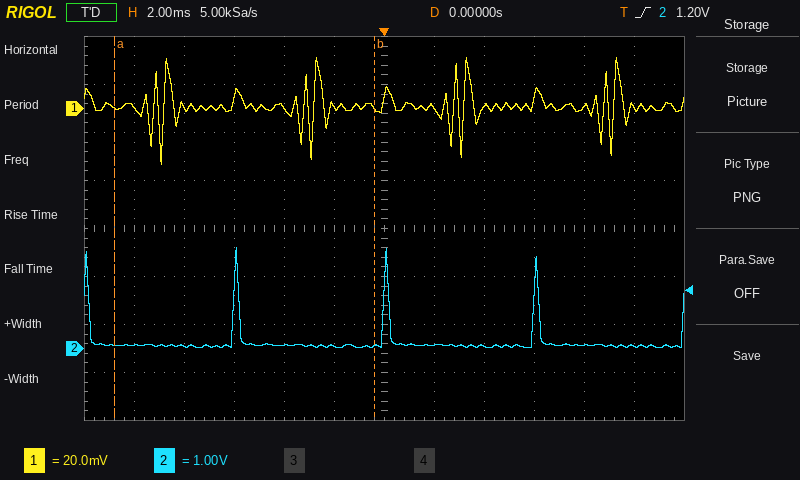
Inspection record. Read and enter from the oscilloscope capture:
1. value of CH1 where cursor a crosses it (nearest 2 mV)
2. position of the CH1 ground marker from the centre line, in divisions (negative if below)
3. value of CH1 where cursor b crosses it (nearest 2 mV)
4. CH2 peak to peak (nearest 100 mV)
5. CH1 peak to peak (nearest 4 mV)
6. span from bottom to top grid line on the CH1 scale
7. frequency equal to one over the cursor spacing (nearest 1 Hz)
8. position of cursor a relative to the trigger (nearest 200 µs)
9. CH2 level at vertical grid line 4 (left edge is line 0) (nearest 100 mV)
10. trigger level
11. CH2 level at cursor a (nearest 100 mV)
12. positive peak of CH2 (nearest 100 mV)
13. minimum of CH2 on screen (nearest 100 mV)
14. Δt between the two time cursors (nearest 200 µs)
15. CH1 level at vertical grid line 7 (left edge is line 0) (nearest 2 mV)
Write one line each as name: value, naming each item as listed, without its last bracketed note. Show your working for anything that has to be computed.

value of CH1 where cursor a crosses it: 0 mV
position of the CH1 ground marker from the centre line, in divisions: +2.5 div
value of CH1 where cursor b crosses it: 0 mV
CH2 peak to peak: 2.1 V − (0.0 V) = 2.1 V
CH1 peak to peak: 44 mV
span from bottom to top grid line on the CH1 scale: 160 mV
frequency equal to one over the cursor spacing: 1 / 10.4 ms ≈ 96 Hz
position of cursor a relative to the trigger: -10.8 ms
CH2 level at vertical grid line 4 (left edge is line 0): 100 mV
trigger level: 1.20 V
CH2 level at cursor a: 100 mV
positive peak of CH2: 2.1 V
minimum of CH2 on screen: 0.0 V
Δt between the two time cursors: 10.4 ms
CH1 level at vertical grid line 7 (left edge is line 0): 0 mV
